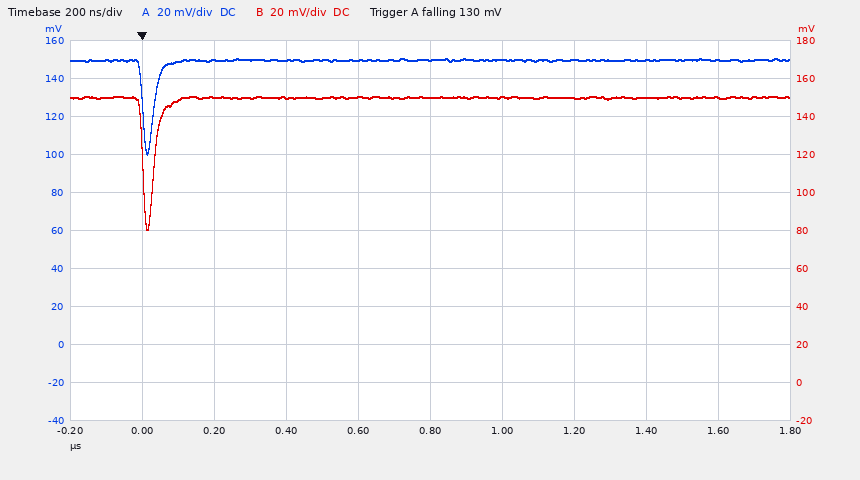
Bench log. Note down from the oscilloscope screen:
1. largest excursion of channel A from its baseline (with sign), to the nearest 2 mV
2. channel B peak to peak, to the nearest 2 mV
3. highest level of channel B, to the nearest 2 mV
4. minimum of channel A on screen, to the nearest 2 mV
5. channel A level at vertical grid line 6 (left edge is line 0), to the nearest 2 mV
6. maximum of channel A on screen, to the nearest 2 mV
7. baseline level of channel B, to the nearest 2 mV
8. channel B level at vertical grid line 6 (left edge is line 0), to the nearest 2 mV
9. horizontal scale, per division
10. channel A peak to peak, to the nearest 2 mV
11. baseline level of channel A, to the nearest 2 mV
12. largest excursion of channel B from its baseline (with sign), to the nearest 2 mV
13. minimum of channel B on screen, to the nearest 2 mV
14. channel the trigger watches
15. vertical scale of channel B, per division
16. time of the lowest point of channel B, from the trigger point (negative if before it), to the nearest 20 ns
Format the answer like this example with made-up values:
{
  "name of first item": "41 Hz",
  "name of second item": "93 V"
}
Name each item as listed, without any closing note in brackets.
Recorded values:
{
  "largest excursion of channel A from its baseline (with sign), to the nearest 2 mV": "-50 mV",
  "channel B peak to peak, to the nearest 2 mV": "70 mV",
  "highest level of channel B, to the nearest 2 mV": "150 mV",
  "minimum of channel A on screen, to the nearest 2 mV": "100 mV",
  "channel A level at vertical grid line 6 (left edge is line 0), to the nearest 2 mV": "150 mV",
  "maximum of channel A on screen, to the nearest 2 mV": "150 mV",
  "baseline level of channel B, to the nearest 2 mV": "150 mV",
  "channel B level at vertical grid line 6 (left edge is line 0), to the nearest 2 mV": "150 mV",
  "horizontal scale, per division": "200 ns",
  "channel A peak to peak, to the nearest 2 mV": "50 mV",
  "baseline level of channel A, to the nearest 2 mV": "150 mV",
  "largest excursion of channel B from its baseline (with sign), to the nearest 2 mV": "-70 mV",
  "minimum of channel B on screen, to the nearest 2 mV": "80 mV",
  "channel the trigger watches": "channel A",
  "vertical scale of channel B, per division": "20 mV",
  "time of the lowest point of channel B, from the trigger point (negative if before it), to the nearest 20 ns": "+20 ns"
}
